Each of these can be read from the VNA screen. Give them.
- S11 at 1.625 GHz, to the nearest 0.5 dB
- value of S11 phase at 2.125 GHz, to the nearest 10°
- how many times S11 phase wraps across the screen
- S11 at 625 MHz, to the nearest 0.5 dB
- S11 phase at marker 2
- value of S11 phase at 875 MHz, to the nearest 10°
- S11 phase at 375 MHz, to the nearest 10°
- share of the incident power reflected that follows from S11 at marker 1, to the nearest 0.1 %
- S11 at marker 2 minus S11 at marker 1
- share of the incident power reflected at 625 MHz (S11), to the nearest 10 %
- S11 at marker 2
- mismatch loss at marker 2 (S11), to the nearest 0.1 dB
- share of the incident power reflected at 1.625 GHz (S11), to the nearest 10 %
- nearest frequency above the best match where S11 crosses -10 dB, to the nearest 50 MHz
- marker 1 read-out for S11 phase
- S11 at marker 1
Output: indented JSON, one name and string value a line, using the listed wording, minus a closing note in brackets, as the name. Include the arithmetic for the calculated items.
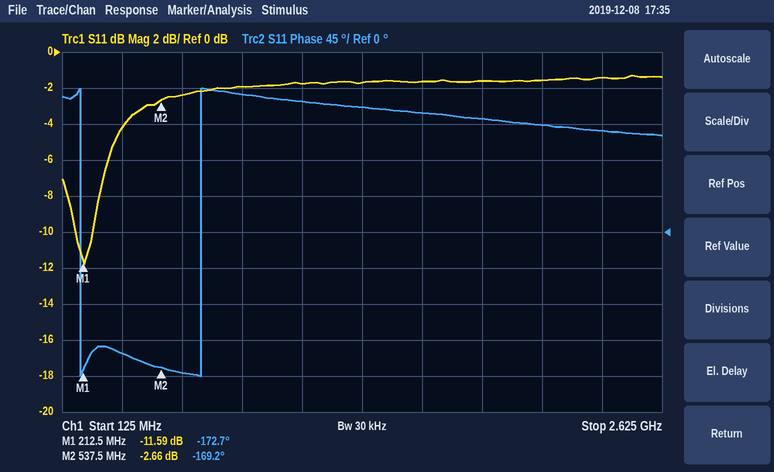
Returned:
{
  "S11 at 1.625 GHz, to the nearest 0.5 dB": "-1.5 dB",
  "value of S11 phase at 2.125 GHz, to the nearest 10°": "130°",
  "how many times S11 phase wraps across the screen": "2",
  "S11 at 625 MHz, to the nearest 0.5 dB": "-2.5 dB",
  "S11 phase at marker 2": "-169.2°",
  "value of S11 phase at 875 MHz, to the nearest 10°": "170°",
  "S11 phase at 375 MHz, to the nearest 10°": "-150°",
  "share of the incident power reflected that follows from S11 at marker 1, to the nearest 0.1 %": "10^(-11.59/10) ≈ 6.9 %",
  "S11 at marker 2 minus S11 at marker 1": "-2.66 − (-11.59) = 8.93 dB",
  "share of the incident power reflected at 625 MHz (S11), to the nearest 10 %": "10^(-2.5/10) ≈ 56.2 %, so 60 % to the nearest 10 %",
  "S11 at marker 2": "-2.66 dB",
  "mismatch loss at marker 2 (S11), to the nearest 0.1 dB": "−10 log10(1 − 10^(-2.66/10)) ≈ 3.4 dB",
  "share of the incident power reflected at 1.625 GHz (S11), to the nearest 10 %": "10^(-1.5/10) ≈ 70.8 %, so 70 % to the nearest 10 %",
  "nearest frequency above the best match where S11 crosses -10 dB, to the nearest 50 MHz": "250 MHz",
  "marker 1 read-out for S11 phase": "-172.7°",
  "S11 at marker 1": "-11.59 dB"
}
